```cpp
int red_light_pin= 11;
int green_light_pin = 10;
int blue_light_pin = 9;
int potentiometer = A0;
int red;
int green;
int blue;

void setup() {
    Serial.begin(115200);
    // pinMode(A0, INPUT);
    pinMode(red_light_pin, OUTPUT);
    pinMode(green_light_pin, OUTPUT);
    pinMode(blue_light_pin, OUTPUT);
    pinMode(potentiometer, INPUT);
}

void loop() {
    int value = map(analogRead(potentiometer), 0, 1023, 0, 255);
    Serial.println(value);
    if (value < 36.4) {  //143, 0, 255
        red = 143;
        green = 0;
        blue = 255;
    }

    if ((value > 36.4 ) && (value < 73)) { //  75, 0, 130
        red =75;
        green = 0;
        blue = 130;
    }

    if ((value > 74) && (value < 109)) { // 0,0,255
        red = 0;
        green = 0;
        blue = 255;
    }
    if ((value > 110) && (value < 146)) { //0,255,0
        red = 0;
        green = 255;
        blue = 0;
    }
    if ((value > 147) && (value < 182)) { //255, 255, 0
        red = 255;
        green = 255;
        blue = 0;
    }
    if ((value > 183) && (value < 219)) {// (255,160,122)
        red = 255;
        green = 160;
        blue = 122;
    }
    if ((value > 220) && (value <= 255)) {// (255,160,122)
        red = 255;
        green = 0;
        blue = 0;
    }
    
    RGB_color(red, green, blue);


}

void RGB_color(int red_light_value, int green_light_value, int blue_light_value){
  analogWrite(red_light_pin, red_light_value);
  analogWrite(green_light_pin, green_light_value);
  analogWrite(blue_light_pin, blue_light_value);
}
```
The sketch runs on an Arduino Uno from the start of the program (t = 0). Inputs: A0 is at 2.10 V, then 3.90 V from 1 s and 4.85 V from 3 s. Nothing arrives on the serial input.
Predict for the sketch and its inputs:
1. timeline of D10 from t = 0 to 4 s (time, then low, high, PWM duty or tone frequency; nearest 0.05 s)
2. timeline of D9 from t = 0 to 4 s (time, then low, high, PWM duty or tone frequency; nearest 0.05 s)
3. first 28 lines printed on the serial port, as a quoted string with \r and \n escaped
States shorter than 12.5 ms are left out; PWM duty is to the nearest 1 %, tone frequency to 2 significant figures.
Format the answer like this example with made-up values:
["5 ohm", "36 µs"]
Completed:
["0 s low; 1 s PWM 63 %; 3 s low", "0 s high; 1 s PWM 48 %; 3 s low", "\"107\\r\\n107\\r\\n107\\r\\n107\\r\\n107\\r\\n107\\r\\n107\\r\\n107\\r\\n107\\r\\n107\\r\\n107\\r\\n107\\r\\n107\\r\\n107\\r\\n107\\r\\n107\\r\\n107\\r\\n107\\r\\n107\\r\\n107\\r\\n107\\r\\n107\\r\\n107\\r\\n107\\r\\n107\\r\\n107\\r\\n107\\r\\n107\\r\\n\""]
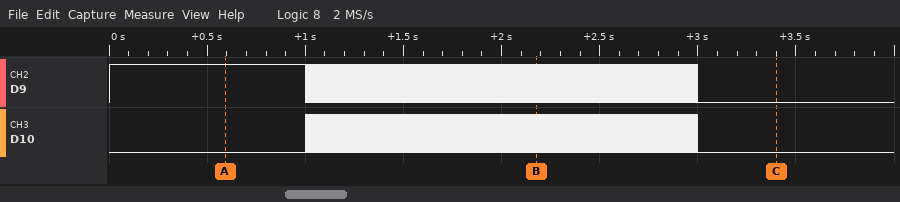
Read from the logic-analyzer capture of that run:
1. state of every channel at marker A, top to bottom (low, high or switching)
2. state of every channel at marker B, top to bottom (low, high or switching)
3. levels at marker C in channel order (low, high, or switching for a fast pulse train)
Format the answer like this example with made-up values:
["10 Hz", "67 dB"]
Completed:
["D9 high, D10 low", "D9 switching, D10 switching", "D9 low, D10 low"]
